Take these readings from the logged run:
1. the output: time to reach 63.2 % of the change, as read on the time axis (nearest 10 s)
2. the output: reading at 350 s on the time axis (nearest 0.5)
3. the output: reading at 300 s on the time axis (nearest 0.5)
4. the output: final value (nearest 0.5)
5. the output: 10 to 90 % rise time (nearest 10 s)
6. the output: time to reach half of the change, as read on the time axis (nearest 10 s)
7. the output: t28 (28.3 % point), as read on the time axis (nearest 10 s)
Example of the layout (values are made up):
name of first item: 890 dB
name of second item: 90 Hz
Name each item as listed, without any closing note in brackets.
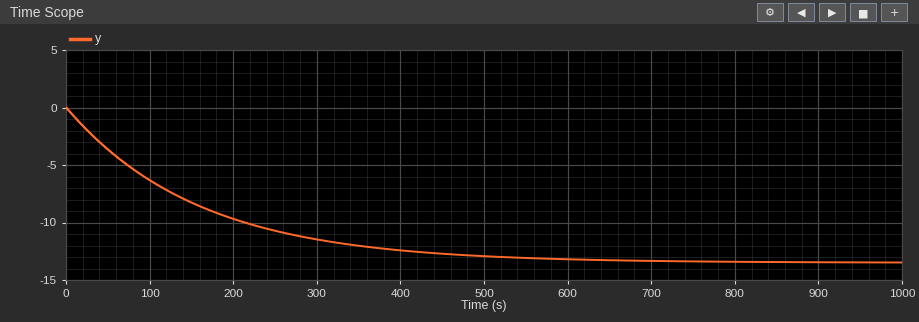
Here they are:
the output: time to reach 63.2 % of the change, as read on the time axis: 160 s
the output: reading at 350 s on the time axis: -12.0
the output: reading at 300 s on the time axis: -11.5
the output: final value: -13.5
the output: 10 to 90 % rise time: 350 s
the output: time to reach half of the change, as read on the time axis: 110 s
the output: t28 (28.3 % point), as read on the time axis: 50 s
